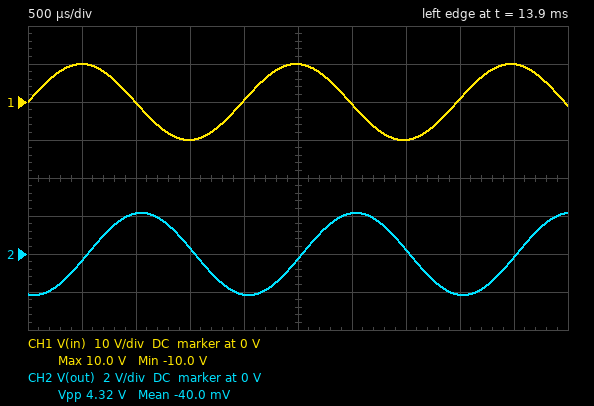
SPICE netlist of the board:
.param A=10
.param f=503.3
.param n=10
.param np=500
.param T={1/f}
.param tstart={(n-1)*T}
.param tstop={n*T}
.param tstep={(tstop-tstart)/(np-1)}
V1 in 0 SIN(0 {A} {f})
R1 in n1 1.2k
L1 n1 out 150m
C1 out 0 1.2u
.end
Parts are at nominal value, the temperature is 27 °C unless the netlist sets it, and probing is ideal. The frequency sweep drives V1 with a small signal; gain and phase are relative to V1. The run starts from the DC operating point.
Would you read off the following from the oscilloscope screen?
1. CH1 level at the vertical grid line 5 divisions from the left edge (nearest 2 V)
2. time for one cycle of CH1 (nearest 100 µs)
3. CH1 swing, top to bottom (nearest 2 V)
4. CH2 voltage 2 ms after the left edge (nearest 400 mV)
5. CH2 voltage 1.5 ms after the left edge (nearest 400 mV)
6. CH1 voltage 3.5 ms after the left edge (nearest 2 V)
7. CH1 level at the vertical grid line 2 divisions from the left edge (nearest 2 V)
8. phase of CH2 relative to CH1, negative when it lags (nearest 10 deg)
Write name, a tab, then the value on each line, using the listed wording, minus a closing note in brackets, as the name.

CH1 level at the vertical grid line 5 divisions from the left edge	10 V
time for one cycle of CH1	2.0 ms
CH1 swing, top to bottom	20 V
CH2 voltage 2 ms after the left edge	-2.0 V
CH2 voltage 1.5 ms after the left edge	400 mV
CH1 voltage 3.5 ms after the left edge	-10 V
CH1 level at the vertical grid line 2 divisions from the left edge	0 V
phase of CH2 relative to CH1, negative when it lags	-100 deg
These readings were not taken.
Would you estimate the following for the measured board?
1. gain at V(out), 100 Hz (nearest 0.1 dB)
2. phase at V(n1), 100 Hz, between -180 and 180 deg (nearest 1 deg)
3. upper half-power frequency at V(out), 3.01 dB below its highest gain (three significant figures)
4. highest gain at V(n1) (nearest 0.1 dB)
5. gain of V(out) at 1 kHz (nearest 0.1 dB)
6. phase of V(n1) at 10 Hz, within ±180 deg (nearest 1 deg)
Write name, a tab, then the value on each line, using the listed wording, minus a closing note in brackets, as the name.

gain at V(out), 100 Hz	-2.3 dB
phase at V(n1), 100 Hz, between -180 and 180 deg	-44 deg
upper half-power frequency at V(out), 3.01 dB below its highest gain	121 Hz
highest gain at V(n1)	0 dB
gain of V(out) at 1 kHz	-20.8 dB
phase of V(n1) at 10 Hz, within ±180 deg	-5 deg
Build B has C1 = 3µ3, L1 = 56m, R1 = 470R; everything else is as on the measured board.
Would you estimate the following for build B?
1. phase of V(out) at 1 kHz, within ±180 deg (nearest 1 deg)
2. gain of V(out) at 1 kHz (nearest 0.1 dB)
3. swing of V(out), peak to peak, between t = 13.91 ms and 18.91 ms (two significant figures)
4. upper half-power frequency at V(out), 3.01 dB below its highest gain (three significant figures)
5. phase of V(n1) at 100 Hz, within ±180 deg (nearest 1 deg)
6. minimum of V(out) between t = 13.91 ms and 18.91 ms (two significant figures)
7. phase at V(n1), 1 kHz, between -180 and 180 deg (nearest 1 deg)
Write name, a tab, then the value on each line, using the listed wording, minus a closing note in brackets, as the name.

phase of V(out) at 1 kHz, within ±180 deg	-123 deg
gain of V(out) at 1 kHz	-21.3 dB
swing of V(out), peak to peak, between t = 13.91 ms and 18.91 ms	4.0 V
upper half-power frequency at V(out), 3.01 dB below its highest gain	111 Hz
phase of V(n1) at 100 Hz, within ±180 deg	-46 deg
minimum of V(out) between t = 13.91 ms and 18.91 ms	-2.0 V
phase at V(n1), 1 kHz, between -180 and 180 deg	57 deg
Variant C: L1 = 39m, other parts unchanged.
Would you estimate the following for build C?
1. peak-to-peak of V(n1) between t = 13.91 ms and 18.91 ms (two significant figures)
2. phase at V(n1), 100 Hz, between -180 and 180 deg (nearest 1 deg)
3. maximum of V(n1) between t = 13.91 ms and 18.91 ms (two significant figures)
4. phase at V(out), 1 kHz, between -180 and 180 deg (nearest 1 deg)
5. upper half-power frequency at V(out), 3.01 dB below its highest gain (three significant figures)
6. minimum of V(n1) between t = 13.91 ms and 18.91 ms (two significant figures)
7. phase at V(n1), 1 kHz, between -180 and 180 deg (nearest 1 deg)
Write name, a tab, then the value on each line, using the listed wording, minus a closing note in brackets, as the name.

peak-to-peak of V(n1) between t = 13.91 ms and 18.91 ms	2.3 V
phase at V(n1), 100 Hz, between -180 and 180 deg	-43 deg
maximum of V(n1) between t = 13.91 ms and 18.91 ms	1.2 V
phase at V(out), 1 kHz, between -180 and 180 deg	-95 deg
upper half-power frequency at V(out), 3.01 dB below its highest gain	113 Hz
minimum of V(n1) between t = 13.91 ms and 18.91 ms	-1.2 V
phase at V(n1), 1 kHz, between -180 and 180 deg	85 deg
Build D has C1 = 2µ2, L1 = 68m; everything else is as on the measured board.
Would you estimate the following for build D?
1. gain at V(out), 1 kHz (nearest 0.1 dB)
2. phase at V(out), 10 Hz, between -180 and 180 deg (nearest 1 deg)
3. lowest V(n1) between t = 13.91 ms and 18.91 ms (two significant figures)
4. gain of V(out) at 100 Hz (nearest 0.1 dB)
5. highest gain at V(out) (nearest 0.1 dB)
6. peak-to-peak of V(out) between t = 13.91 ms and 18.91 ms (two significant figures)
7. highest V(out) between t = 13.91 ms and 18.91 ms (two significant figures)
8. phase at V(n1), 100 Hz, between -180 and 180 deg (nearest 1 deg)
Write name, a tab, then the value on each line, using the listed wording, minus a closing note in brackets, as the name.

gain at V(out), 1 kHz	-24.8 dB
phase at V(out), 10 Hz, between -180 and 180 deg	-9 deg
lowest V(n1) between t = 13.91 ms and 18.91 ms	-590 mV
gain of V(out) at 100 Hz	-5.6 dB
highest gain at V(out)	0 dB
peak-to-peak of V(out) between t = 13.91 ms and 18.91 ms	2.4 V
highest V(out) between t = 13.91 ms and 18.91 ms	1.2 V
phase at V(n1), 100 Hz, between -180 and 180 deg	-60 deg
